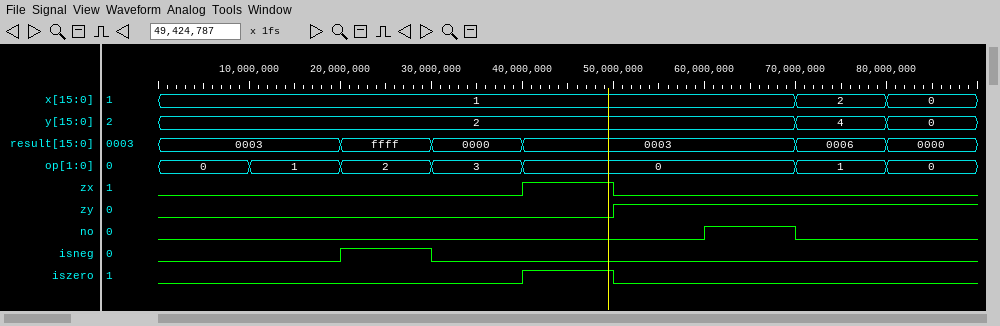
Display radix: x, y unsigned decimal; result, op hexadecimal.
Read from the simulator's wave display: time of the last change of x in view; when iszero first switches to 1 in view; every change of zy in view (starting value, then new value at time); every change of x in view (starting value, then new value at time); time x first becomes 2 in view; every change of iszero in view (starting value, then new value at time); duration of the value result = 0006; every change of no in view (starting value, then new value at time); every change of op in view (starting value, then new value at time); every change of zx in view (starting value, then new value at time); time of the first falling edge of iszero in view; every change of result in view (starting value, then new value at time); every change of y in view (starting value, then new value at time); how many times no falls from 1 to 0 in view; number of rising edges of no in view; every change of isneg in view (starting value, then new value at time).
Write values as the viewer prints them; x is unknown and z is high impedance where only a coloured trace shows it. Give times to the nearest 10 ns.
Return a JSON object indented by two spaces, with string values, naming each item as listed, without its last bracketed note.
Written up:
{
  "time of the last change of x in view": "80 ns",
  "when iszero first switches to 1 in view": "40 ns",
  "every change of zy in view": "0, 1 at 50 ns",
  "every change of x in view": "1, 2 at 70 ns, 0 at 80 ns",
  "time x first becomes 2 in view": "70 ns",
  "every change of iszero in view": "0, 1 at 40 ns, 0 at 50 ns",
  "duration of the value result = 0006": "10 ns",
  "every change of no in view": "0, 1 at 60 ns, 0 at 70 ns",
  "every change of op in view": "0, 1 at 10 ns, 2 at 20 ns, 3 at 30 ns, 0 at 40 ns, 1 at 70 ns, 0 at 80 ns",
  "every change of zx in view": "0, 1 at 40 ns, 0 at 50 ns",
  "time of the first falling edge of iszero in view": "50 ns",
  "every change of result in view": "0003, ffff at 20 ns, 0000 at 30 ns, 0003 at 40 ns, 0006 at 70 ns, 0000 at 80 ns",
  "every change of y in view": "2, 4 at 70 ns, 0 at 80 ns",
  "how many times no falls from 1 to 0 in view": "1",
  "number of rising edges of no in view": "1",
  "every change of isneg in view": "0, 1 at 20 ns, 0 at 30 ns"
}
